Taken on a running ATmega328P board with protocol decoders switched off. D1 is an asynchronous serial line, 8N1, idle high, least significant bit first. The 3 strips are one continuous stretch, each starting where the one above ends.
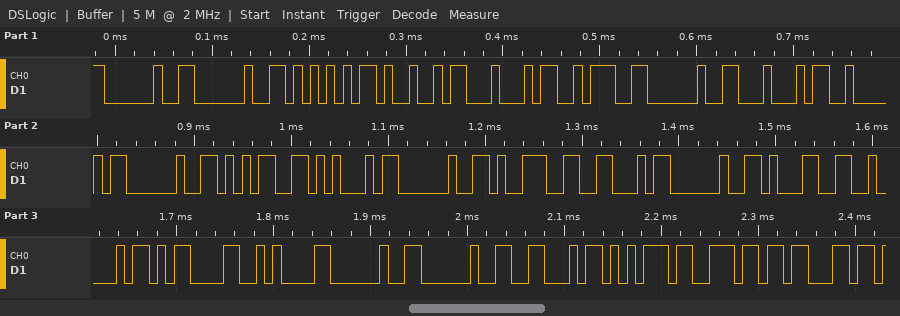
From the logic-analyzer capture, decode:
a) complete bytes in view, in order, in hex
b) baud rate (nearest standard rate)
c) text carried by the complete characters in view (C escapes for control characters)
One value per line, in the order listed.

20 20 55 49 44 3A 20 44 42 20 35 45 20 39 46 20 31 42 0D 0A 20 20 46 75 6E 63
115200 baud
"  UID: DB 5E 9F 1B\r\n  Func"
